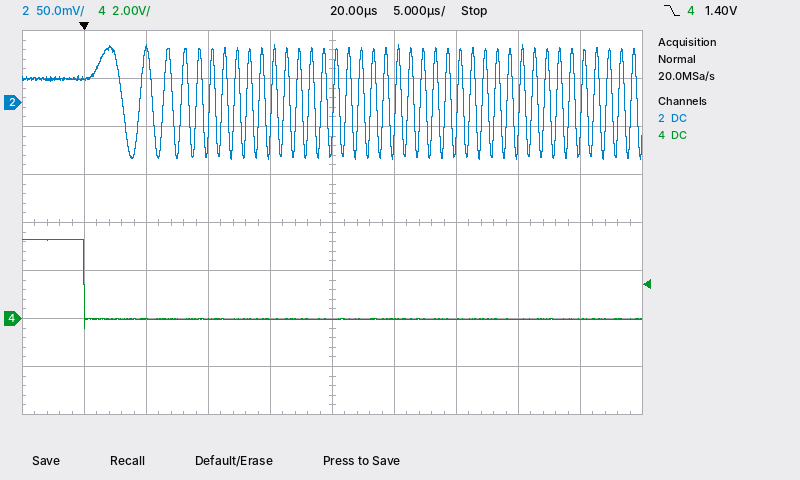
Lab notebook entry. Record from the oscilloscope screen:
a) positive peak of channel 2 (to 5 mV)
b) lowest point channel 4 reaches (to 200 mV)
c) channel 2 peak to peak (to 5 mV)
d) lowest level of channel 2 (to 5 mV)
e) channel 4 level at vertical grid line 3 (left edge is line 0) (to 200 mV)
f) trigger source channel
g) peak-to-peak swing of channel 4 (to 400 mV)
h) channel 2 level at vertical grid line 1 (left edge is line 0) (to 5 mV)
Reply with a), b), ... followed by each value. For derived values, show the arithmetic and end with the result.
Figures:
a) 60 mV
b) -400 mV
c) 60 mV − (-60 mV) = 120 mV
d) -60 mV
e) 0.0 V
f) channel 4
g) 3.6 V
h) 25 mV
